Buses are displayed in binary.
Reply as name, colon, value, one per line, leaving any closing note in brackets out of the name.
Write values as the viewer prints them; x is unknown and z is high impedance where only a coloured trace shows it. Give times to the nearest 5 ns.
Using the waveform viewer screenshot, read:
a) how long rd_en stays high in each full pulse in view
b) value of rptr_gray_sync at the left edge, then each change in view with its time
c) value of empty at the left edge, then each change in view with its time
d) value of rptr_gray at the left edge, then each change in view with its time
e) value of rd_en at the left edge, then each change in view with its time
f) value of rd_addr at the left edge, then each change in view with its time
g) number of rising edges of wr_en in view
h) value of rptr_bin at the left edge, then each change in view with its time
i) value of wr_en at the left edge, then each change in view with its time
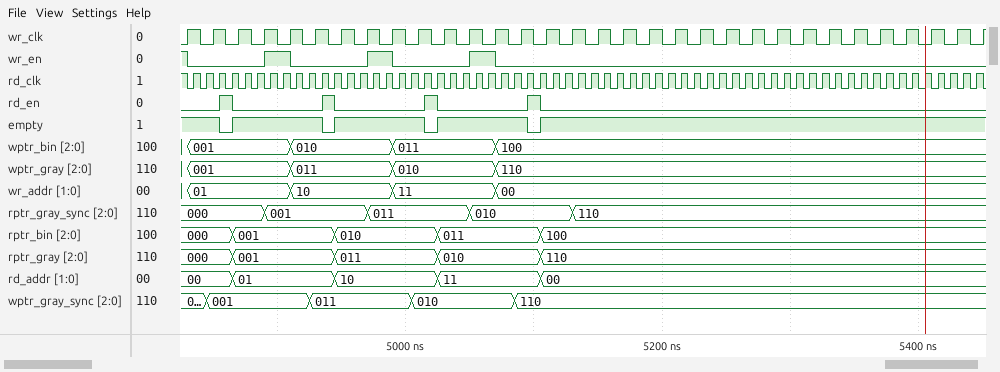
how long rd_en stays high in each full pulse in view: 10 ns, 10 ns, 10 ns, 10 ns
value of rptr_gray_sync at the left edge, then each change in view with its time: 000, 001 at 4890 ns, 011 at 4970 ns, 010 at 5050 ns, 110 at 5130 ns
value of empty at the left edge, then each change in view with its time: 1, 0 at 4855 ns, 1 at 4865 ns, 0 at 4935 ns, 1 at 4945 ns, 0 at 5015 ns, 1 at 5025 ns, 0 at 5095 ns, 1 at 5105 ns
value of rptr_gray at the left edge, then each change in view with its time: 000, 001 at 4865 ns, 011 at 4945 ns, 010 at 5025 ns, 110 at 5105 ns
value of rd_en at the left edge, then each change in view with its time: 0, 1 at 4855 ns, 0 at 4865 ns, 1 at 4935 ns, 0 at 4945 ns, 1 at 5015 ns, 0 at 5025 ns, 1 at 5095 ns, 0 at 5105 ns
value of rd_addr at the left edge, then each change in view with its time: 00, 01 at 4865 ns, 10 at 4945 ns, 11 at 5025 ns, 00 at 5105 ns
number of rising edges of wr_en in view: 3
value of rptr_bin at the left edge, then each change in view with its time: 000, 001 at 4865 ns, 010 at 4945 ns, 011 at 5025 ns, 100 at 5105 ns
value of wr_en at the left edge, then each change in view with its time: 1, 0 at 4830 ns, 1 at 4890 ns, 0 at 4910 ns, 1 at 4970 ns, 0 at 4990 ns, 1 at 5050 ns, 0 at 5070 ns
